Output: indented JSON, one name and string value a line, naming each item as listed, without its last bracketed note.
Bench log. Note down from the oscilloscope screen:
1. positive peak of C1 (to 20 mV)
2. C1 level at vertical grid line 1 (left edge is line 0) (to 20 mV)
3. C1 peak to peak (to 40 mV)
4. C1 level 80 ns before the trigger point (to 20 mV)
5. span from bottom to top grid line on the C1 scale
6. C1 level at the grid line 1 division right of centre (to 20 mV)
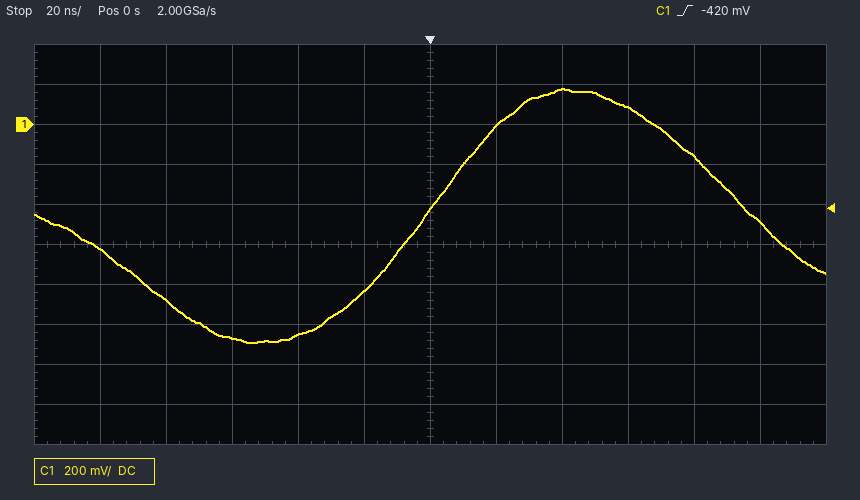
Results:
{
  "positive peak of C1": "180 mV",
  "C1 level at vertical grid line 1 (left edge is line 0)": "-620 mV",
  "C1 peak to peak": "1.28 V",
  "C1 level 80 ns before the trigger point": "-880 mV",
  "span from bottom to top grid line on the C1 scale": "2 V",
  "C1 level at the grid line 1 division right of centre": "0 mV"
}
